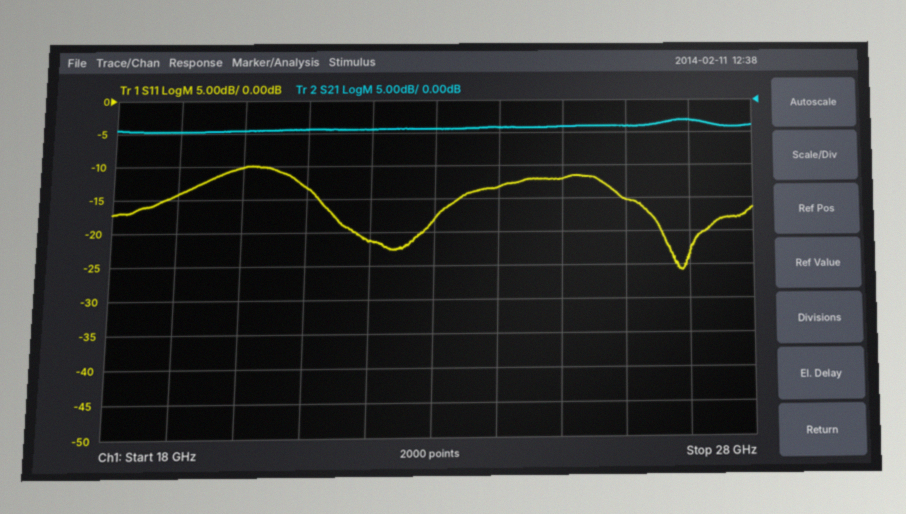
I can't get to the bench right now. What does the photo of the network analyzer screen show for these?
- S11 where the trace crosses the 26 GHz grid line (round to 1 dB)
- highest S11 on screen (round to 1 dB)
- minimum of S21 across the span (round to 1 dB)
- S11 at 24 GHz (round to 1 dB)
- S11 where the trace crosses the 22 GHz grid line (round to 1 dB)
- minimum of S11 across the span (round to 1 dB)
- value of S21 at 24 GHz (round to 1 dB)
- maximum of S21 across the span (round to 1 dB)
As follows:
-15 dB
-10 dB
-5 dB
-13 dB
-21 dB
-26 dB
-4 dB
-3 dB
